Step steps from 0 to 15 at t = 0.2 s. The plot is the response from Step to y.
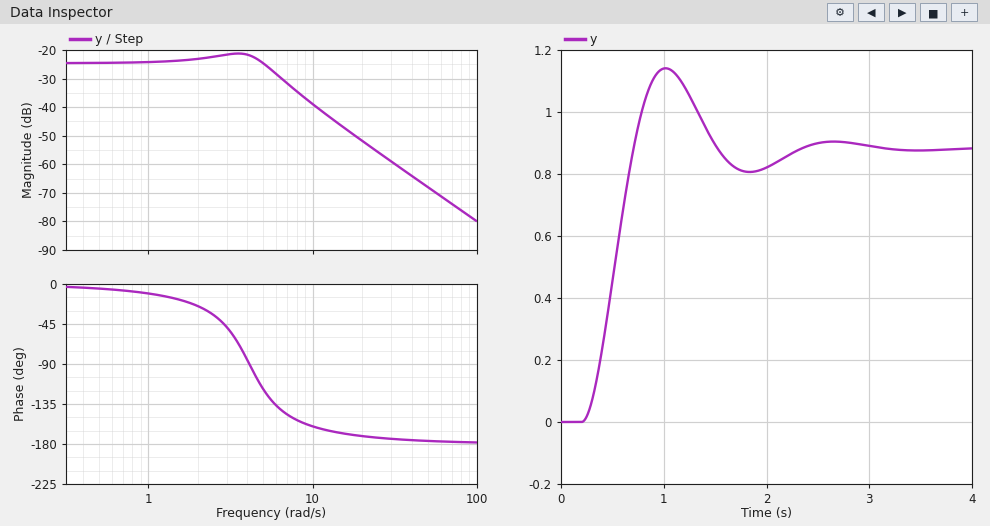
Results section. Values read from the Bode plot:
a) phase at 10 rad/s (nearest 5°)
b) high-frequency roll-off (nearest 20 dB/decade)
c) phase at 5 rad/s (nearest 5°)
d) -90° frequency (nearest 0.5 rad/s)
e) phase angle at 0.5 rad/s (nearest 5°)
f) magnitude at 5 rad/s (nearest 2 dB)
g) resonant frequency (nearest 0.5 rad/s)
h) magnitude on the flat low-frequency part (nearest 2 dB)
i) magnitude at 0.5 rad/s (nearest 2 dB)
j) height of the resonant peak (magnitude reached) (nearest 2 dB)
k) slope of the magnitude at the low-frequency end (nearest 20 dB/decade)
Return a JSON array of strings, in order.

["-160°", "-40 dB/decade", "-120°", "4.0 rad/s", "-5°", "-24 dB", "3.5 rad/s", "-24 dB", "-24 dB", "-22 dB", "0 dB/decade"]
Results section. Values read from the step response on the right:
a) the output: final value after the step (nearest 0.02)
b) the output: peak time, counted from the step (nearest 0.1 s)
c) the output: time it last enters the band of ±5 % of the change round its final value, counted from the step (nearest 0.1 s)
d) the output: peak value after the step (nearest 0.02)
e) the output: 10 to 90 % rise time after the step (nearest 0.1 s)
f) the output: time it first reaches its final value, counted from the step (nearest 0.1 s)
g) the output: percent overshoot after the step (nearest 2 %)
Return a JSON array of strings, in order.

["0.88", "0.8 s", "1.9 s", "1.14", "0.3 s", "0.5 s", "30 %"]
